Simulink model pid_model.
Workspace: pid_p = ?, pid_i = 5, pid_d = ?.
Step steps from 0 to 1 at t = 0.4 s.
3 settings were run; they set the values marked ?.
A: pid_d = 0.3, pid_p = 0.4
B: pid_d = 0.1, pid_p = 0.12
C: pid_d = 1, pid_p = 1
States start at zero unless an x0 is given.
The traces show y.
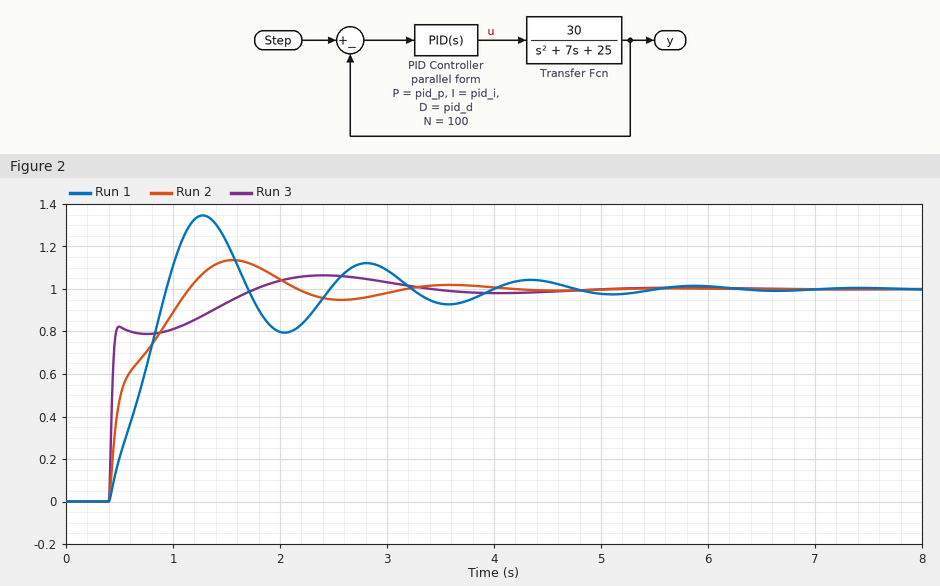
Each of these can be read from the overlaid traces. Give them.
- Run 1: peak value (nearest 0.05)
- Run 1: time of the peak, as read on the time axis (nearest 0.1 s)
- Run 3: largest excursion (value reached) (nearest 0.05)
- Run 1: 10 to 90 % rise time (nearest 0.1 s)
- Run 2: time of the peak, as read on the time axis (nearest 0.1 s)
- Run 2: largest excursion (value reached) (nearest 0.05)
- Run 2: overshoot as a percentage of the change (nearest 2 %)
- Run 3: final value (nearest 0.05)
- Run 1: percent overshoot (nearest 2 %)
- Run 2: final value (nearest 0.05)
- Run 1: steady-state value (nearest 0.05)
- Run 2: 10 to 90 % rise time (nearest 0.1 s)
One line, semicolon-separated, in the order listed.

1.35; 1.3 s; 1.05; 0.4 s; 1.6 s; 1.15; 14 %; 1.00; 34 %; 1.00; 1.00; 0.6 s
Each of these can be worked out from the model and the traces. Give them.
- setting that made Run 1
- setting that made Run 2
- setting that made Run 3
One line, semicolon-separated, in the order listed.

B; A; C
